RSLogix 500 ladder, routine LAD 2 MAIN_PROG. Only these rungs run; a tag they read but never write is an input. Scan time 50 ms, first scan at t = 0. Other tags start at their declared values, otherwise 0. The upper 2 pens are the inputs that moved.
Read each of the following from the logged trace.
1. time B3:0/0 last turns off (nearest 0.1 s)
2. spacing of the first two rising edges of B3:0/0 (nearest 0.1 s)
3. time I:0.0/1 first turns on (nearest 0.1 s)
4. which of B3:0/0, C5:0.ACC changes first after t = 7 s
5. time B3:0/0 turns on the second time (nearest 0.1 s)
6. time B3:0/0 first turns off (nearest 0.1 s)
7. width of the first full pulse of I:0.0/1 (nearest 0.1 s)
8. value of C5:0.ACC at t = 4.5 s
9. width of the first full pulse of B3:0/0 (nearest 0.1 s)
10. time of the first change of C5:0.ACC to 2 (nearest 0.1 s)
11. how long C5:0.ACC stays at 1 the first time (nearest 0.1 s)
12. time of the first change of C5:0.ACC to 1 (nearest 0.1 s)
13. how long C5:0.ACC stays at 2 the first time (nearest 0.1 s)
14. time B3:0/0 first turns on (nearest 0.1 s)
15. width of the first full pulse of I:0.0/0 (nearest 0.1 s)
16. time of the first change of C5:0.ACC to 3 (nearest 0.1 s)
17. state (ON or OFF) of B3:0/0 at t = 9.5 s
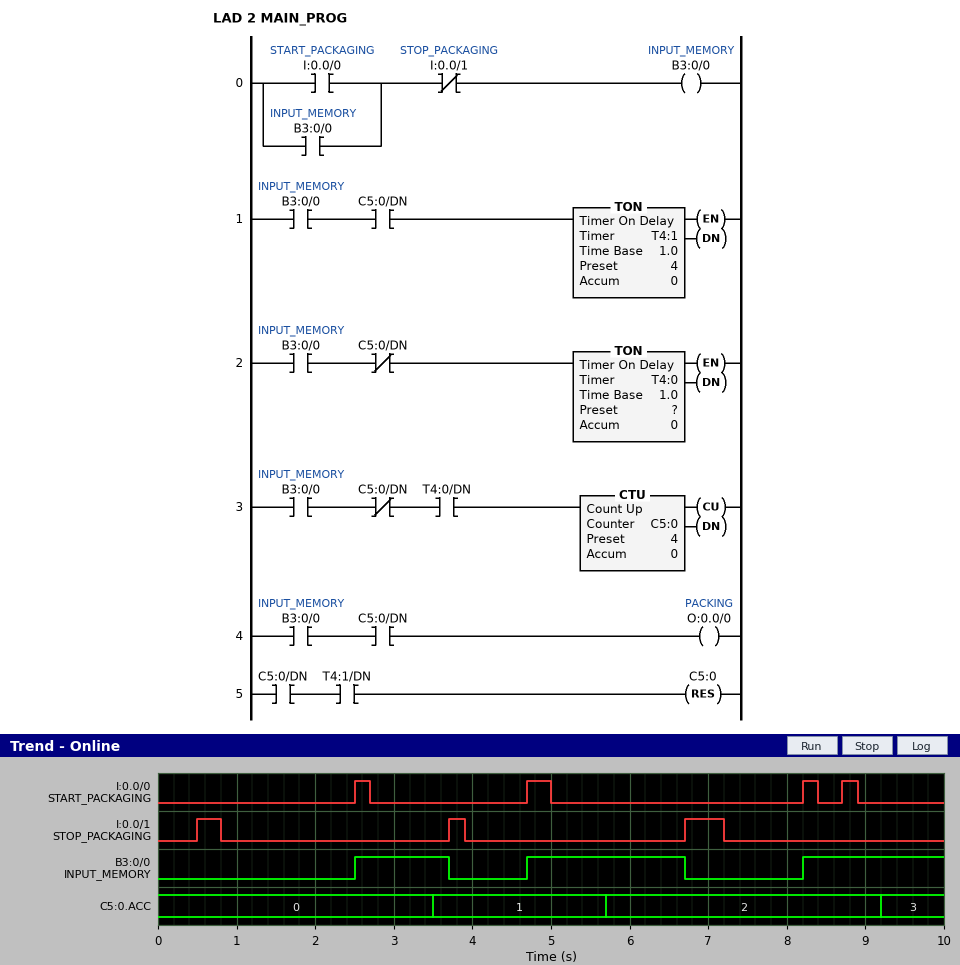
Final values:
6.7 s
2.2 s
0.5 s
B3:0/0
4.7 s
3.7 s
0.3 s
1
1.2 s
5.7 s
2.2 s
3.5 s
3.5 s
2.5 s
0.2 s
9.2 s
ON
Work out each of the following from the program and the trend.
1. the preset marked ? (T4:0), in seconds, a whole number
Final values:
1 s
